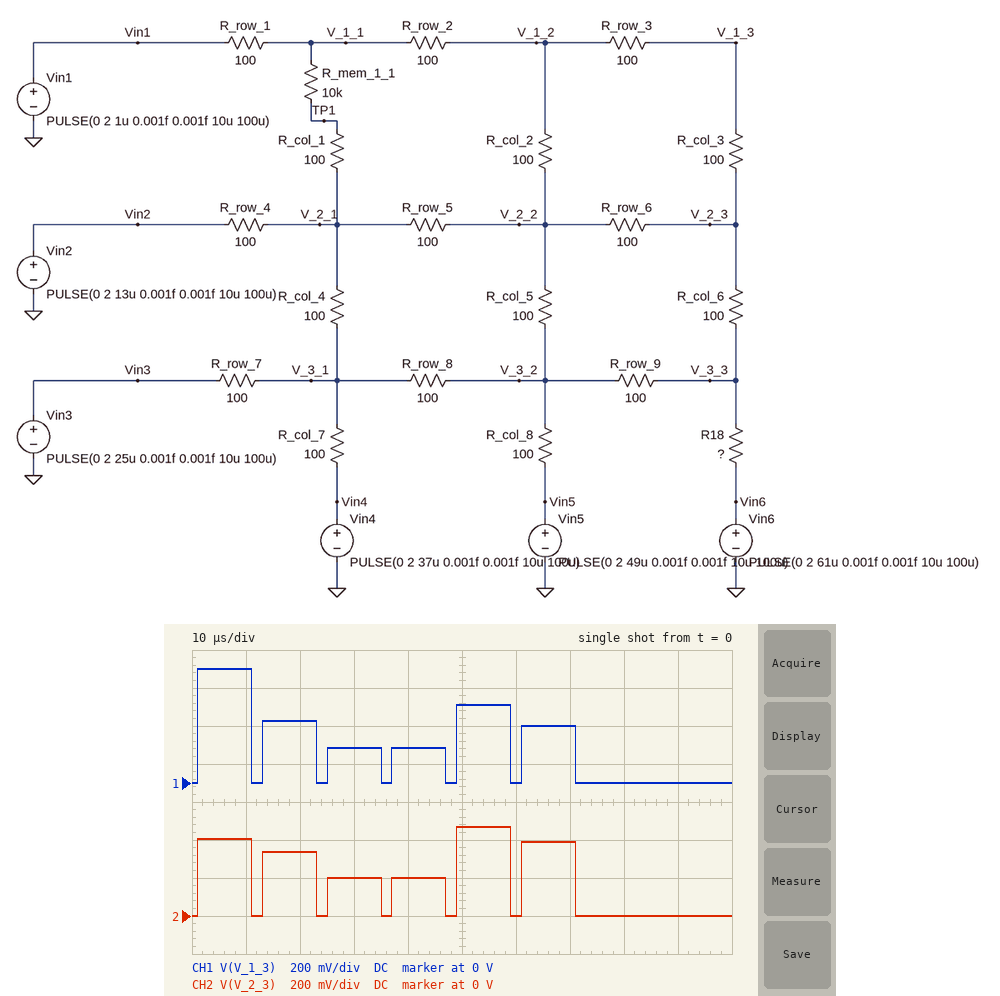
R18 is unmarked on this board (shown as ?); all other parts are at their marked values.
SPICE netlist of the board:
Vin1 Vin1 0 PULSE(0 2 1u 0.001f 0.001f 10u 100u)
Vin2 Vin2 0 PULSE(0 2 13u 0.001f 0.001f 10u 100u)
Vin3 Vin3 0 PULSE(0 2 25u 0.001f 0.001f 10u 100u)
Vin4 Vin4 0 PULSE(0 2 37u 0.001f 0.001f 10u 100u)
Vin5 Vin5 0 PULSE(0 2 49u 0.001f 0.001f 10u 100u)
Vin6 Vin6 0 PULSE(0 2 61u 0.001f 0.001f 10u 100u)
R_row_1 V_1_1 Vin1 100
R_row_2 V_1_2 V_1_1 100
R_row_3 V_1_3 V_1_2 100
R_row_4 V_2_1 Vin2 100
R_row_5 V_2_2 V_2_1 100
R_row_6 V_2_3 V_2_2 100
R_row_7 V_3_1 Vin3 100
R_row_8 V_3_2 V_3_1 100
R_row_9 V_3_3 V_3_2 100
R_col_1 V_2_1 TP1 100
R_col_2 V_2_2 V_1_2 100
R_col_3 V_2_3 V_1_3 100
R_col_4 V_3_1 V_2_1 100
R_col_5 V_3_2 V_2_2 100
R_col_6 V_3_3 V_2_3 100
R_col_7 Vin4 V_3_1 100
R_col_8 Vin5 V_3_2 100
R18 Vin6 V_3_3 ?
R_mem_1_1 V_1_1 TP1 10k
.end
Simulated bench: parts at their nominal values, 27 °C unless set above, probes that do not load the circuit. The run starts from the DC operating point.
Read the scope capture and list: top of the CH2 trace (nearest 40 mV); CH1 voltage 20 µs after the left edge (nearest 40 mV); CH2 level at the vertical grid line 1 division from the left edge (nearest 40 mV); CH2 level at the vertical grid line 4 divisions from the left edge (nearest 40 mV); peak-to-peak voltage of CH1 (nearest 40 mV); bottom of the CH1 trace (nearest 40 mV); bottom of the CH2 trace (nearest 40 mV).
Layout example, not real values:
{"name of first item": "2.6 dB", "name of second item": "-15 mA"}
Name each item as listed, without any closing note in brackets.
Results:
{"top of the CH2 trace": "480 mV", "CH1 voltage 20 µs after the left edge": "320 mV", "CH2 level at the vertical grid line 1 division from the left edge": "400 mV", "CH2 level at the vertical grid line 4 divisions from the left edge": "200 mV", "peak-to-peak voltage of CH1": "600 mV", "bottom of the CH1 trace": "0 V", "bottom of the CH2 trace": "0 V"}
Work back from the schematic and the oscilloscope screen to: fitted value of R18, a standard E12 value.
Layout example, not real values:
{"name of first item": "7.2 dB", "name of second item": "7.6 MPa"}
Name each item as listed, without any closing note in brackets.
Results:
{"fitted value of R18, a standard E12 value": "220 Ω"}
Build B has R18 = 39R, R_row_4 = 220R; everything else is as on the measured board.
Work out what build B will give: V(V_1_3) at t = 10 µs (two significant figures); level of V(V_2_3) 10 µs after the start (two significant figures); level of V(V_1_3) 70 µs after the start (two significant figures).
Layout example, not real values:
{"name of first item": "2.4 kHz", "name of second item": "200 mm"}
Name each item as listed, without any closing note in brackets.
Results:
{"V(V_1_3) at t = 10 µs": "540 mV", "level of V(V_2_3) 10 µs after the start": "330 mV", "level of V(V_1_3) 70 µs after the start": "720 mV"}
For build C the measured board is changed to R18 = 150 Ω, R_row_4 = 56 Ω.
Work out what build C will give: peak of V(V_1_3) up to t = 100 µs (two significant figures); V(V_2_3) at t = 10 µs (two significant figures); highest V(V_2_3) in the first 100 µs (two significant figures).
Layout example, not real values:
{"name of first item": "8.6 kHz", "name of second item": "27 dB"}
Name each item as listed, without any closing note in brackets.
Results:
{"peak of V(V_1_3) up to t = 100 µs": "570 mV", "V(V_2_3) at t = 10 µs": "370 mV", "highest V(V_2_3) in the first 100 µs": "480 mV"}
